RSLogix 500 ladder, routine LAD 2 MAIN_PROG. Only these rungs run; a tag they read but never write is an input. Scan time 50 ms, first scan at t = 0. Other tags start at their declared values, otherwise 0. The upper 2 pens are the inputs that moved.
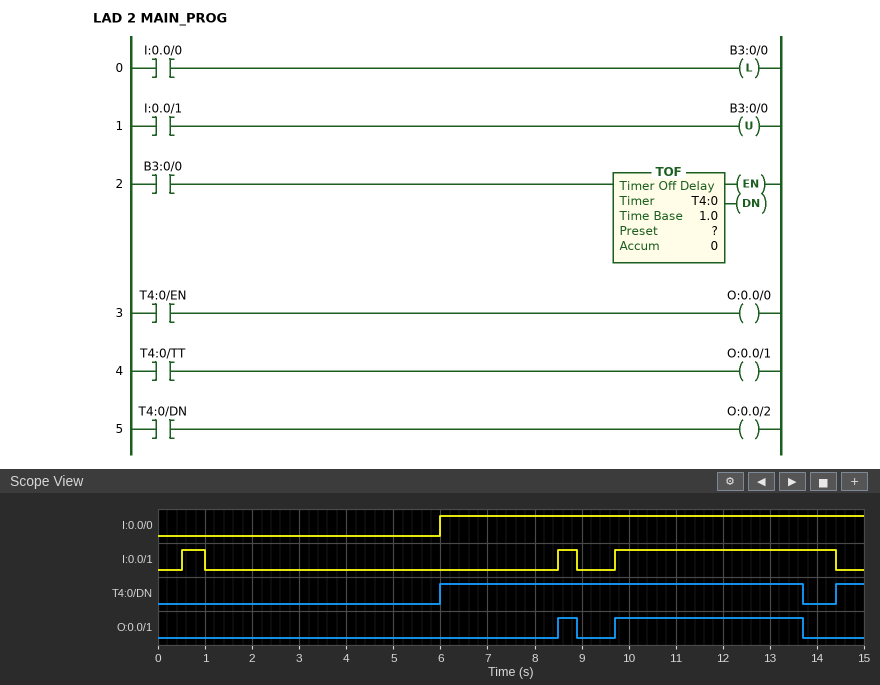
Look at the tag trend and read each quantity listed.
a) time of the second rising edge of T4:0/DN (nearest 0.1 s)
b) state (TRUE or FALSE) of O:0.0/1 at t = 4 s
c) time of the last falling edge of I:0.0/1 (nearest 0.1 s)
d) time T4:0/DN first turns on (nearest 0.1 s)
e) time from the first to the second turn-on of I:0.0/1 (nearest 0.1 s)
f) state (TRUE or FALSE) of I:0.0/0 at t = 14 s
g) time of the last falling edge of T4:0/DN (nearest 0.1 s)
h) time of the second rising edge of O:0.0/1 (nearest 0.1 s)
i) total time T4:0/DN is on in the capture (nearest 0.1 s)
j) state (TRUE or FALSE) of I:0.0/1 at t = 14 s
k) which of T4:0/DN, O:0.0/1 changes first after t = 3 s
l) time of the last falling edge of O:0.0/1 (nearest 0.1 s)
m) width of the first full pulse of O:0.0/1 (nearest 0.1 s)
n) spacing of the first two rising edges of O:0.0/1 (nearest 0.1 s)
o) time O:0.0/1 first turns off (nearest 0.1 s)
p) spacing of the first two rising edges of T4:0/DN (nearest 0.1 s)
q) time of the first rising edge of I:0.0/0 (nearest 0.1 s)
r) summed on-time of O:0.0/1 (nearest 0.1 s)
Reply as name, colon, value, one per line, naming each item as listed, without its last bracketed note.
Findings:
time of the second rising edge of T4:0/DN: 14.4 s
state (TRUE or FALSE) of O:0.0/1 at t = 4 s: FALSE
time of the last falling edge of I:0.0/1: 14.4 s
time T4:0/DN first turns on: 6.0 s
time from the first to the second turn-on of I:0.0/1: 8.0 s
state (TRUE or FALSE) of I:0.0/0 at t = 14 s: TRUE
time of the last falling edge of T4:0/DN: 13.7 s
time of the second rising edge of O:0.0/1: 9.7 s
total time T4:0/DN is on in the capture: 8.3 s
state (TRUE or FALSE) of I:0.0/1 at t = 14 s: TRUE
which of T4:0/DN, O:0.0/1 changes first after t = 3 s: T4:0/DN
time of the last falling edge of O:0.0/1: 13.7 s
width of the first full pulse of O:0.0/1: 0.4 s
spacing of the first two rising edges of O:0.0/1: 1.2 s
time O:0.0/1 first turns off: 8.9 s
spacing of the first two rising edges of T4:0/DN: 8.4 s
time of the first rising edge of I:0.0/0: 6.0 s
summed on-time of O:0.0/1: 4.4 s
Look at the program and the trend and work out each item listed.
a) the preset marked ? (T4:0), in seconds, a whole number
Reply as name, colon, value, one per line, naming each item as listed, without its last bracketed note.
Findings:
the preset marked ? (T4:0), in seconds, a whole number: 4 s
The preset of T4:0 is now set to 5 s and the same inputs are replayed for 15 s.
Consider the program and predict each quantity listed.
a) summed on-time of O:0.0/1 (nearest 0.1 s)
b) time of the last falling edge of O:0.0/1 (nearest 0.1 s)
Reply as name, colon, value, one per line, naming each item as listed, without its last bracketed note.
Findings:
summed on-time of O:0.0/1: 5.1 s
time of the last falling edge of O:0.0/1: 14.4 s
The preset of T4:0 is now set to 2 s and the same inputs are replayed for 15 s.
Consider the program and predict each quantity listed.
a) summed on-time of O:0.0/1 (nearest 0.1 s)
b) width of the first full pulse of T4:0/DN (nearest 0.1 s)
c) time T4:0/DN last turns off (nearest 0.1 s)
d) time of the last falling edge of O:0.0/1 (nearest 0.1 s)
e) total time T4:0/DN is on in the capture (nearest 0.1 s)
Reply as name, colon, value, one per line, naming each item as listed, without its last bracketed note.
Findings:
summed on-time of O:0.0/1: 2.4 s
width of the first full pulse of T4:0/DN: 5.7 s
time T4:0/DN last turns off: 11.7 s
time of the last falling edge of O:0.0/1: 11.7 s
total time T4:0/DN is on in the capture: 6.3 s
